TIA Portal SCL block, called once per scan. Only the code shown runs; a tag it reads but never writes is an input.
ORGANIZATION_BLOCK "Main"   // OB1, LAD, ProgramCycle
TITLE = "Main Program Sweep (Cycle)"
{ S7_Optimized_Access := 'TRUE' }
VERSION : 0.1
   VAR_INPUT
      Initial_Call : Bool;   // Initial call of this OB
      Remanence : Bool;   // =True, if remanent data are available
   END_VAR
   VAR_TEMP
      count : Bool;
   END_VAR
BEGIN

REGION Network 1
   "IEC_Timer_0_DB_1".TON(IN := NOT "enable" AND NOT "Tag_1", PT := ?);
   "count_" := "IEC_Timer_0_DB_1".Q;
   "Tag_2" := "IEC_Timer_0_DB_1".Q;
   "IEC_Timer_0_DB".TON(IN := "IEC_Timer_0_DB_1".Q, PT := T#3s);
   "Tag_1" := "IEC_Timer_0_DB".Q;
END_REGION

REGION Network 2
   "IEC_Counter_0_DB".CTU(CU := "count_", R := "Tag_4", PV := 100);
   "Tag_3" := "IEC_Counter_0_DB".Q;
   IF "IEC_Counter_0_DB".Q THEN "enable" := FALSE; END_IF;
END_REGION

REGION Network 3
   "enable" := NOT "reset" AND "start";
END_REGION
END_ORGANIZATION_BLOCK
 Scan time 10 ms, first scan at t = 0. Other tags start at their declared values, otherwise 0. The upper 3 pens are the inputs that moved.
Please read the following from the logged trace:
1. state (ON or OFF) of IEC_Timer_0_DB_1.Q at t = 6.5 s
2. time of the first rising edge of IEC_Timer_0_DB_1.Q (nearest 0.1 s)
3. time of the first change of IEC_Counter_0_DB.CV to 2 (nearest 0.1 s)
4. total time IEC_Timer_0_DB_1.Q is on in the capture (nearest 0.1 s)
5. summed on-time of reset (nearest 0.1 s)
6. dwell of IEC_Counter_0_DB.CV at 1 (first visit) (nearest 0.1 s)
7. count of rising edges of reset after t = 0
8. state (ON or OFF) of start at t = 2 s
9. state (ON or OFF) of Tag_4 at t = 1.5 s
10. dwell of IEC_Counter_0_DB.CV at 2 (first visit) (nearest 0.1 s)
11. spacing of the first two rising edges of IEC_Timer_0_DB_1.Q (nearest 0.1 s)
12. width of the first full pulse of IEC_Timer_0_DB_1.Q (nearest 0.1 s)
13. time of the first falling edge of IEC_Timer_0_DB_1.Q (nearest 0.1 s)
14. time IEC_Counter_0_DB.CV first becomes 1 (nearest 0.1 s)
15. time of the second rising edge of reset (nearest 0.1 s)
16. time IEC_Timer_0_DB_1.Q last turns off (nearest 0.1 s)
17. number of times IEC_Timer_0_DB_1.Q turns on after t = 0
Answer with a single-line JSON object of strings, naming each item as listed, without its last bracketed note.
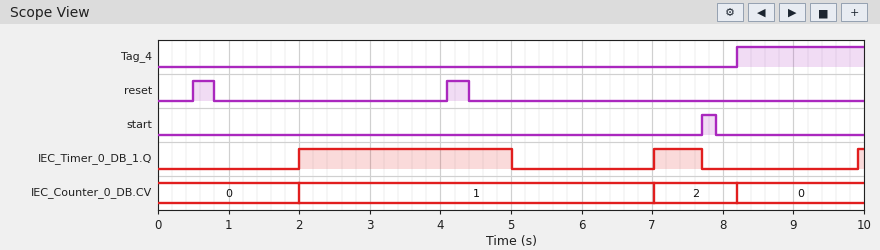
{"state (ON or OFF) of IEC_Timer_0_DB_1.Q at t = 6.5 s": "OFF", "time of the first rising edge of IEC_Timer_0_DB_1.Q": "2.0 s", "time of the first change of IEC_Counter_0_DB.CV to 2": "7.0 s", "total time IEC_Timer_0_DB_1.Q is on in the capture": "3.8 s", "summed on-time of reset": "0.6 s", "dwell of IEC_Counter_0_DB.CV at 1 (first visit)": "5.0 s", "count of rising edges of reset after t = 0": "2", "state (ON or OFF) of start at t = 2 s": "OFF", "state (ON or OFF) of Tag_4 at t = 1.5 s": "OFF", "dwell of IEC_Counter_0_DB.CV at 2 (first visit)": "1.2 s", "spacing of the first two rising edges of IEC_Timer_0_DB_1.Q": "5.0 s", "width of the first full pulse of IEC_Timer_0_DB_1.Q": "3.0 s", "time of the first falling edge of IEC_Timer_0_DB_1.Q": "5.0 s", "time IEC_Counter_0_DB.CV first becomes 1": "2.0 s", "time of the second rising edge of reset": "4.1 s", "time IEC_Timer_0_DB_1.Q last turns off": "7.7 s", "number of times IEC_Timer_0_DB_1.Q turns on after t = 0": "3"}
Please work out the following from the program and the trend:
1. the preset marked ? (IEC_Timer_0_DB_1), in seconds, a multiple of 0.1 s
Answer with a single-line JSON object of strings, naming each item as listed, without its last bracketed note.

{"the preset marked ? (IEC_Timer_0_DB_1), in seconds, a multiple of 0.1 s": "2.0 s"}
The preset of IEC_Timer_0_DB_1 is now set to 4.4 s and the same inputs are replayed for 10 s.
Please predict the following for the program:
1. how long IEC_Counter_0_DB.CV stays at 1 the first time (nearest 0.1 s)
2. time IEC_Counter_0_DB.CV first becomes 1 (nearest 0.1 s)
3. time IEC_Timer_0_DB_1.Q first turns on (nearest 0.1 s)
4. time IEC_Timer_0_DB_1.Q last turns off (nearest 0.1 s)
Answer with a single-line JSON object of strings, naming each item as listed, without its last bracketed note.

{"how long IEC_Counter_0_DB.CV stays at 1 the first time": "3.8 s", "time IEC_Counter_0_DB.CV first becomes 1": "4.4 s", "time IEC_Timer_0_DB_1.Q first turns on": "4.4 s", "time IEC_Timer_0_DB_1.Q last turns off": "7.4 s"}
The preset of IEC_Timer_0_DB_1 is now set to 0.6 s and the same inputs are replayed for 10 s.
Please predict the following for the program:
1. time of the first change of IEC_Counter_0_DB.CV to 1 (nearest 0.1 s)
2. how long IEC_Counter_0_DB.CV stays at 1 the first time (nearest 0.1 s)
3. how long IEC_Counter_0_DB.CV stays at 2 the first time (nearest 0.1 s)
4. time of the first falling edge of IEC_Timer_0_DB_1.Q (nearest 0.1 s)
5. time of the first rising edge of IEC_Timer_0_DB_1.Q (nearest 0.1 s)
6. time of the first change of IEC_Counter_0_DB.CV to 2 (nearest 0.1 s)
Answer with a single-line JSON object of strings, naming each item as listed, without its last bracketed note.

{"time of the first change of IEC_Counter_0_DB.CV to 1": "0.6 s", "how long IEC_Counter_0_DB.CV stays at 1 the first time": "3.6 s", "how long IEC_Counter_0_DB.CV stays at 2 the first time": "4.0 s", "time of the first falling edge of IEC_Timer_0_DB_1.Q": "3.6 s", "time of the first rising edge of IEC_Timer_0_DB_1.Q": "0.6 s", "time of the first change of IEC_Counter_0_DB.CV to 2": "4.2 s"}
